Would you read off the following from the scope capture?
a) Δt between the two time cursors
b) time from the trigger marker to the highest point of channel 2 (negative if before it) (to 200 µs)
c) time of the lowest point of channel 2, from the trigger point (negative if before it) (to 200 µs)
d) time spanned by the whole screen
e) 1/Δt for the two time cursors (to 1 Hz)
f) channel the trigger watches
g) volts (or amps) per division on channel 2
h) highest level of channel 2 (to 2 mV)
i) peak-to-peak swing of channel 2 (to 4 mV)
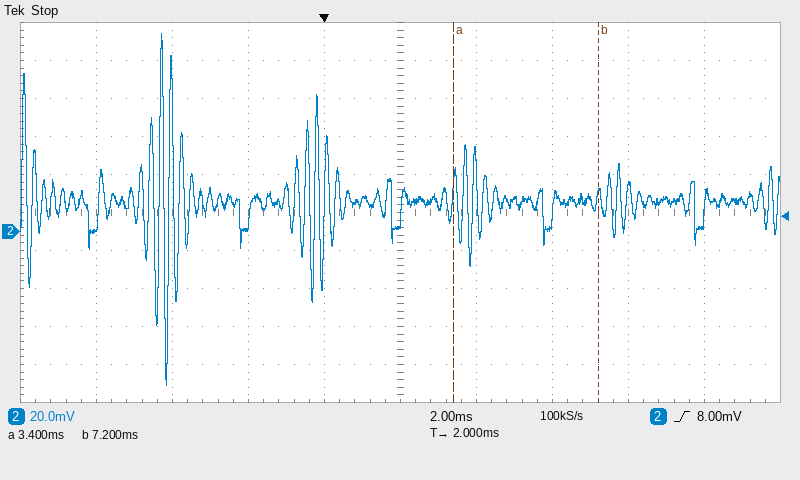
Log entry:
3.8 ms
-4.2 ms
-4.2 ms
20 ms
263 Hz
channel 2
20 mV
104 mV
184 mV
